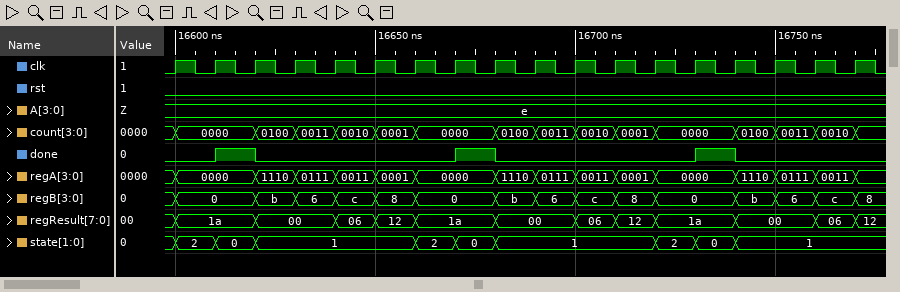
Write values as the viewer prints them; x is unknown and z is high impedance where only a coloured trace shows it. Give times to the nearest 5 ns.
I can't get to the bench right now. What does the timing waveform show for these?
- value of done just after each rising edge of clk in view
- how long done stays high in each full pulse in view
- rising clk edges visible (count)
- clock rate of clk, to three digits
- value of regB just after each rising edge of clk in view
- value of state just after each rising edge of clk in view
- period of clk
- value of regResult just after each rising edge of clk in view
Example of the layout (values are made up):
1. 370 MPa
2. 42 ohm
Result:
1. 0 1 0 0 0 0 0 1 0 0 0 0 0 1 0 0 0 0
2. 10 ns, 10 ns, 10 ns
3. 18
4. 100 MHz
5. 0, 0, b, 6, c, 8, 0, 0, b, 6, c, 8, 0, 0, b, 6, c, 8
6. 2, 0, 1, 1, 1, 1, 2, 0, 1, 1, 1, 1, 2, 0, 1, 1, 1, 1
7. 10 ns
8. 1a, 1a, 00, 00, 06, 12, 1a, 1a, 00, 00, 06, 12, 1a, 1a, 00, 00, 06, 12
